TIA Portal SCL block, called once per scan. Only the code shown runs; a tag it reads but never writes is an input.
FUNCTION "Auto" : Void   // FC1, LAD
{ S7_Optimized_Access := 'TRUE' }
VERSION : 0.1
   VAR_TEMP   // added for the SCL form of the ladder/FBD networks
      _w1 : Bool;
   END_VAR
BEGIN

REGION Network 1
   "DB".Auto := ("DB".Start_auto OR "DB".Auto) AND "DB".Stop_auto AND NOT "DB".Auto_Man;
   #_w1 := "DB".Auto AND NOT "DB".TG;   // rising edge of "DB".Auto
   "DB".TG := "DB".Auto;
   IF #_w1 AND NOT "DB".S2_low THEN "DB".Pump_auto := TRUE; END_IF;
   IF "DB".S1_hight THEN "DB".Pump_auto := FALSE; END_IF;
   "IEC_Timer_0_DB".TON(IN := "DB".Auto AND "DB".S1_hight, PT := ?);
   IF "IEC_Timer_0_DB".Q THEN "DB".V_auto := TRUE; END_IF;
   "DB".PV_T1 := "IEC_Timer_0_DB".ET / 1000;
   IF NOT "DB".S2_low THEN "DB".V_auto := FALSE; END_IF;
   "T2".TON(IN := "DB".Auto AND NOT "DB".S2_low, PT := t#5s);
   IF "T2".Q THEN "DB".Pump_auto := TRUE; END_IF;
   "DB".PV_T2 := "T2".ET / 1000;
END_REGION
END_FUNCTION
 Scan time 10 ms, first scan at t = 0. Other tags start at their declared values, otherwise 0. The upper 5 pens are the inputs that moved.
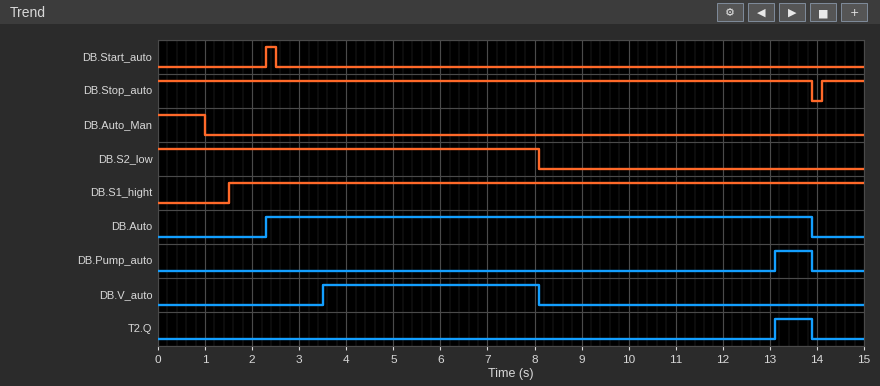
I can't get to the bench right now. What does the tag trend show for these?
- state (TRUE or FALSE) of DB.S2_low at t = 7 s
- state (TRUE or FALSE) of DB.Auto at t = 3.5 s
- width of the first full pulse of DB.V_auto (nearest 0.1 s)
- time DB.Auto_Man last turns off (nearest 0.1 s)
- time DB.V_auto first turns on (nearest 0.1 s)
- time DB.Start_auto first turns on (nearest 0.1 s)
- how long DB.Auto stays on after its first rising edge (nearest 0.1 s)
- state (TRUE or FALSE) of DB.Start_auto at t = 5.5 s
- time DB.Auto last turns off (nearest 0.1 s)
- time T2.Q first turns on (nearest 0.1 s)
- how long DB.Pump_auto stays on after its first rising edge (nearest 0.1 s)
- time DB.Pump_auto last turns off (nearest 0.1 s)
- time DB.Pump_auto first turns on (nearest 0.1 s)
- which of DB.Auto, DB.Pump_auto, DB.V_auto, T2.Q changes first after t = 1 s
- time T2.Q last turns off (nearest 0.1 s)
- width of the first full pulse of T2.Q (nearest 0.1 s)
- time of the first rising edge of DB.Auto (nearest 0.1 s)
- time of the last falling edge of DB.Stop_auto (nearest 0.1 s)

TRUE
TRUE
4.6 s
1.0 s
3.5 s
2.3 s
11.6 s
FALSE
13.9 s
13.1 s
0.8 s
13.9 s
13.1 s
DB.Auto
13.9 s
0.8 s
2.3 s
13.9 s
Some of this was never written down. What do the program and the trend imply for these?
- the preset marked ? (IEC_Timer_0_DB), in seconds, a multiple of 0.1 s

1.2 s
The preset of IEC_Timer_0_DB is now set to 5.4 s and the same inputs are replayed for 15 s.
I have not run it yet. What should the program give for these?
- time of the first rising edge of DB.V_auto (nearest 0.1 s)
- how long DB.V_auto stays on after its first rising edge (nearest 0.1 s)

7.7 s
0.4 s
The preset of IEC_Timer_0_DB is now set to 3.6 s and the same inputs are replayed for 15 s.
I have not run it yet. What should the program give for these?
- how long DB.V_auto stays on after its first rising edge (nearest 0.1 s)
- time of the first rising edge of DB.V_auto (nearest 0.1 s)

2.2 s
5.9 s
